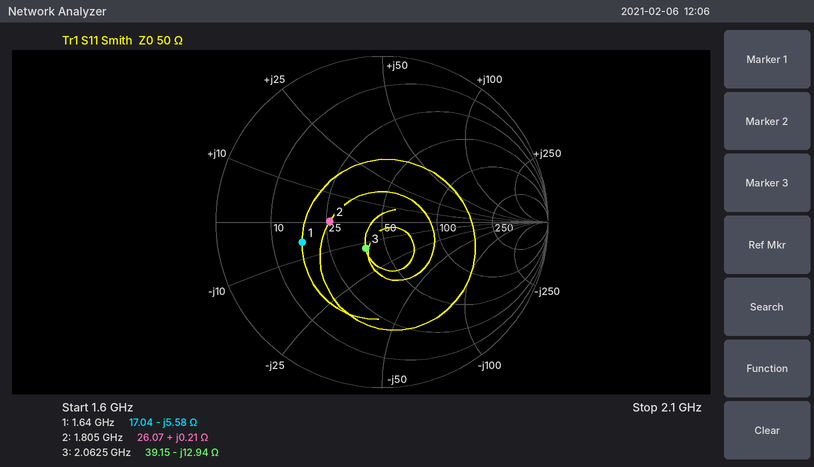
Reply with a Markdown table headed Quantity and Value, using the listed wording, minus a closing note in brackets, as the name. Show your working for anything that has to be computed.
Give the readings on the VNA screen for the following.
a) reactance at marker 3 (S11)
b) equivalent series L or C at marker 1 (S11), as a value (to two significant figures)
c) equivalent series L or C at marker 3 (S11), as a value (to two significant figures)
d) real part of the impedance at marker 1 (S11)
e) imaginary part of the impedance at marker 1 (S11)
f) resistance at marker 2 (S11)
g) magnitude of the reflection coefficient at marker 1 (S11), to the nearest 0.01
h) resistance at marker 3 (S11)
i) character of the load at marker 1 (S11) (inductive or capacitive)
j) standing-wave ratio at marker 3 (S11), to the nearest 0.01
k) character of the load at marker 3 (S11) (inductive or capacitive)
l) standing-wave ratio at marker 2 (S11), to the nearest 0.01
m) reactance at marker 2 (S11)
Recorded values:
| Quantity | Value |
|---|---|
| reactance at marker 3 | -12.94 Ω |
| equivalent series L or C at marker 1 (S11), as a value | C = 1/(2π × 1.64 GHz × 5.58 Ω) ≈ 17 pF |
| equivalent series L or C at marker 3 (S11), as a value | C = 1/(2π × 2.0625 GHz × 12.94 Ω) ≈ 6.0 pF |
| real part of the impedance at marker 1 | 17.04 Ω |
| imaginary part of the impedance at marker 1 | -5.58 Ω |
| resistance at marker 2 | 26.07 Ω |
| magnitude of the reflection coefficient at marker 1 (S11), to the nearest 0.01 | 0.50 |
| resistance at marker 3 | 39.15 Ω |
| character of the load at marker 1 (S11) | capacitive |
| standing-wave ratio at marker 3 (S11), to the nearest 0.01 | 1.46 |
| character of the load at marker 3 (S11) | capacitive |
| standing-wave ratio at marker 2 (S11), to the nearest 0.01 | 1.92 |
| reactance at marker 2 | +0.21 Ω |
